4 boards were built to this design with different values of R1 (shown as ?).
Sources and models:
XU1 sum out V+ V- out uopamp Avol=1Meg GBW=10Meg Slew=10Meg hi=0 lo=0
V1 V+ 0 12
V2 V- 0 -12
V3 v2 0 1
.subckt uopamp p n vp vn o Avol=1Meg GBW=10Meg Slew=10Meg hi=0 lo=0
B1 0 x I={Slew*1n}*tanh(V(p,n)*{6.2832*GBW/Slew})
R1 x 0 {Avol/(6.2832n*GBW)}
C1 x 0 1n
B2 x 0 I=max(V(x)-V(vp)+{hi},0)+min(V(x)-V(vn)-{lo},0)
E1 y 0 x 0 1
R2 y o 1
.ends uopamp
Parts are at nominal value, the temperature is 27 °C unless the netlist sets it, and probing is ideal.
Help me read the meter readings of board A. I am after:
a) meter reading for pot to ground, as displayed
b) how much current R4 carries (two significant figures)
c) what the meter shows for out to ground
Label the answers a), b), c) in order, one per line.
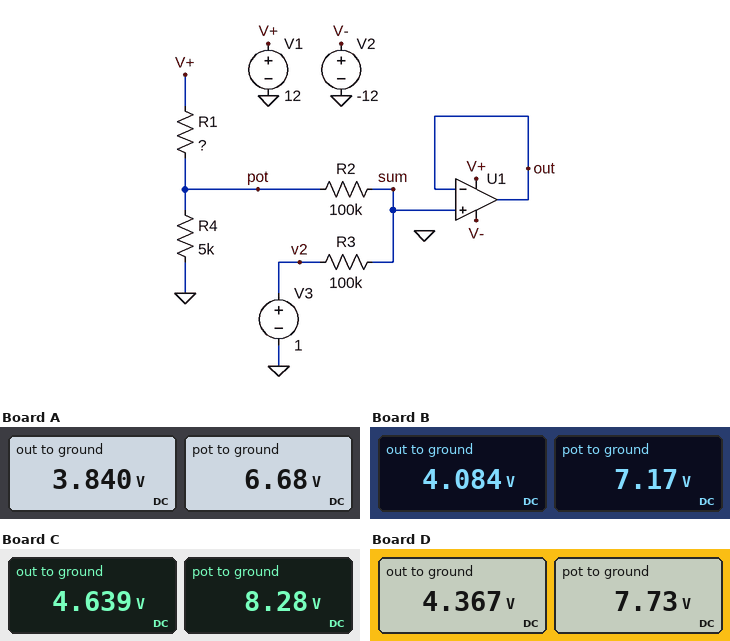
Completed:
a) 6.68 V
b) 1.3 mA
c) 3.840 V
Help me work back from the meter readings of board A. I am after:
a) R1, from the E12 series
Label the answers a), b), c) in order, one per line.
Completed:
a) 3.9 kΩ
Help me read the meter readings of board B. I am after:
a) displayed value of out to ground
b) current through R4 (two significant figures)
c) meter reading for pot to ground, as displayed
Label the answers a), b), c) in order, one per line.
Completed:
a) 4.084 V
b) 1.4 mA
c) 7.17 V
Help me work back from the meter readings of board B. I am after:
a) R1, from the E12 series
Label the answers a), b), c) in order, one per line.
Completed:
a) 3.3 kΩ
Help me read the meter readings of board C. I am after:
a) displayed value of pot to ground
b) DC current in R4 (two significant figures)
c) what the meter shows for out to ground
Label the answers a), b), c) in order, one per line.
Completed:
a) 8.28 V
b) 1.7 mA
c) 4.639 V
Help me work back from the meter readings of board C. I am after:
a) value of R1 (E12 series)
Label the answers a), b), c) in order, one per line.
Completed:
a) 2.2 kΩ
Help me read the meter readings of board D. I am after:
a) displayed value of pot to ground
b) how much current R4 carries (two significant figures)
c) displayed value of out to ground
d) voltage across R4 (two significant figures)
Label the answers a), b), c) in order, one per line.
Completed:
a) 7.73 V
b) 1.5 mA
c) 4.367 V
d) 7.7 V
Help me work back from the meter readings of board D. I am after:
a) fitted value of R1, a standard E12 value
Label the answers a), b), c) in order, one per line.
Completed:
a) 2.7 kΩ
